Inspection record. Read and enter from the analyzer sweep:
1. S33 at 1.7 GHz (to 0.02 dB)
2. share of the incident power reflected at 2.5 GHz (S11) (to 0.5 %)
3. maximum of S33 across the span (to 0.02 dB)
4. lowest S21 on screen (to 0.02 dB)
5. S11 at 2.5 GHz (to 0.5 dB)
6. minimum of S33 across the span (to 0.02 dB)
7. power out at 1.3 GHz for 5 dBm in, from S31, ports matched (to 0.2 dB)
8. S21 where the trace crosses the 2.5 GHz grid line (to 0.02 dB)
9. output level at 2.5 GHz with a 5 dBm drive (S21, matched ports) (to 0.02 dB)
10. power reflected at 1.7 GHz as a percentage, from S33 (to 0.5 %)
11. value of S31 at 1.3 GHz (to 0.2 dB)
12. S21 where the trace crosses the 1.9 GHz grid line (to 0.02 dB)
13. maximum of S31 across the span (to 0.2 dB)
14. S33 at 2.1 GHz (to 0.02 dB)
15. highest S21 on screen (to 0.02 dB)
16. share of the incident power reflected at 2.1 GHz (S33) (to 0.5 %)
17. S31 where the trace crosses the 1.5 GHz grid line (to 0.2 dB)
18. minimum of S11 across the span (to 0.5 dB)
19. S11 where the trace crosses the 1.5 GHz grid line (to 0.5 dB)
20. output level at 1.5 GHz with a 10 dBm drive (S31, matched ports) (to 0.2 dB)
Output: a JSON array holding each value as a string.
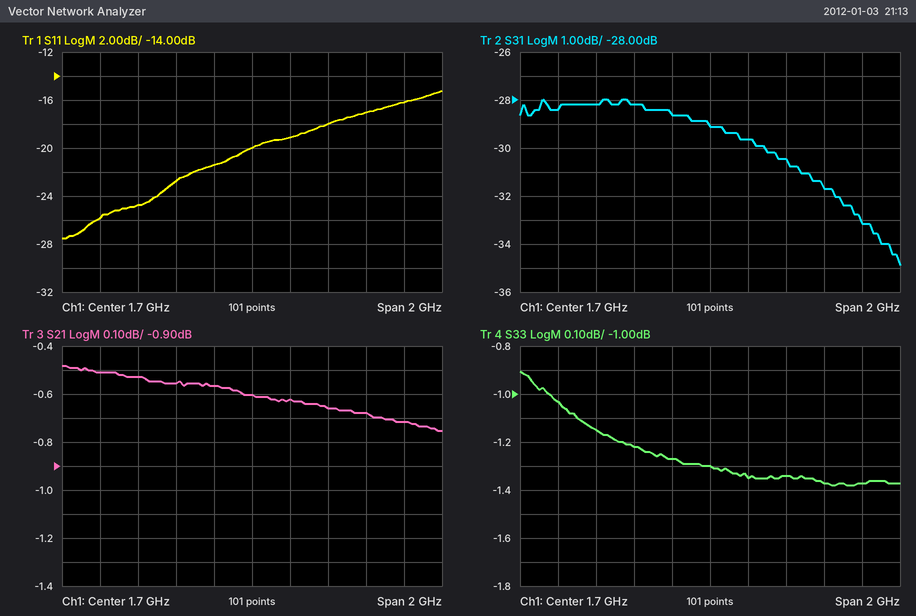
["-1.30 dB", "2.5 %", "-0.90 dB", "-0.76 dB", "-16.0 dB", "-1.38 dB", "-23.2 dBm", "-0.72 dB", "4.28 dBm", "74.0 %", "-28.2 dB", "-0.62 dB", "-28.0 dB", "-1.34 dB", "-0.48 dB", "73.5 %", "-28.6 dB", "-27.5 dB", "-21.5 dB", "-18.6 dBm"]
